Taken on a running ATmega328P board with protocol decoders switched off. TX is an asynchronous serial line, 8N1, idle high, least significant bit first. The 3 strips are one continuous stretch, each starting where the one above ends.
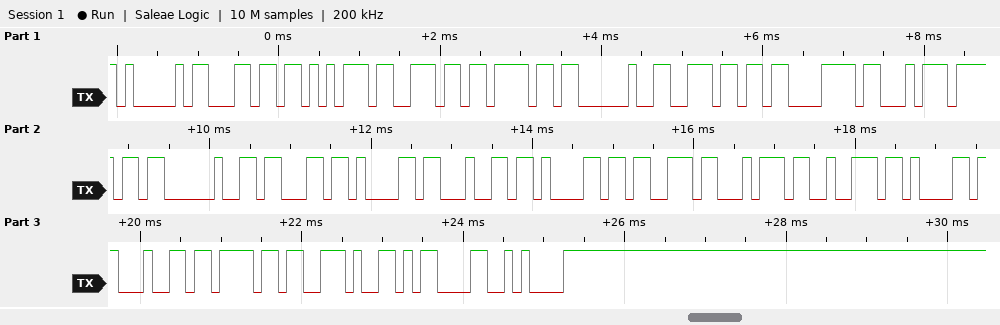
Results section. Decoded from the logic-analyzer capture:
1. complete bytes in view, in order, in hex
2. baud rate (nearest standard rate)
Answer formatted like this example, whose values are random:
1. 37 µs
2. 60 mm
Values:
1. 41 6C 75 6E 6F 20 6E C3 A3 6F 20 63 61 64 61 73 74 72 61 64 6F 2E 0D 0A
2. 9600 baud
